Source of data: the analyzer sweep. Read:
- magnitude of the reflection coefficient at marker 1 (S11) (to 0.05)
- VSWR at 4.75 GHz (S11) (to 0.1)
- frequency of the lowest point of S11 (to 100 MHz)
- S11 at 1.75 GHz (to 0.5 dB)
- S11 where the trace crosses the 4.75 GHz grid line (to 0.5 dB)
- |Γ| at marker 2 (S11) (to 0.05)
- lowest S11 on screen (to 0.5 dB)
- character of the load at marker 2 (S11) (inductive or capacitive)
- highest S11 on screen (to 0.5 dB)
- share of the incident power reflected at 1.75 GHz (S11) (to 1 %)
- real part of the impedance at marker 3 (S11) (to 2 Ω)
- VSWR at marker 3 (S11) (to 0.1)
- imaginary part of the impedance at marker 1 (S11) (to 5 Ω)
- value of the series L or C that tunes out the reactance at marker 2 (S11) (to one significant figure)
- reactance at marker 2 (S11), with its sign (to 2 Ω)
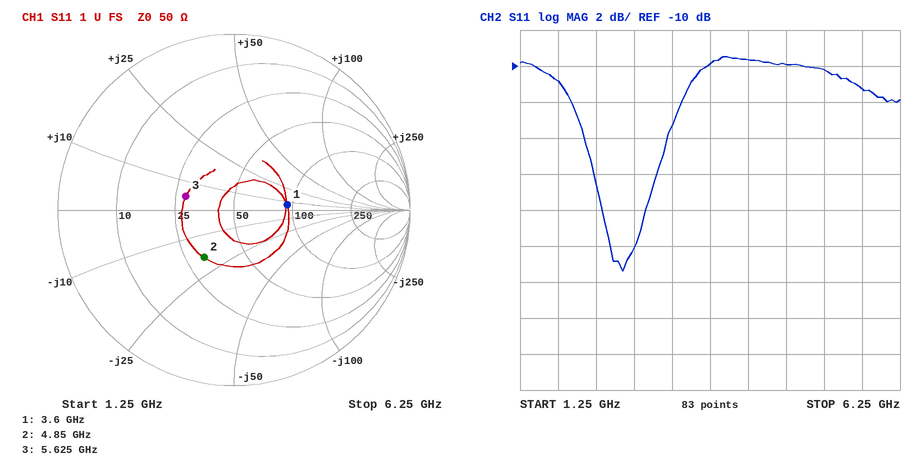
0.30
1.9
2.6 GHz
-11.0 dB
-10.0 dB
0.30
-21.5 dB
capacitive
-9.5 dB
8 %
28 Ω
1.8
+5 Ω
600 pH
-18 Ω
